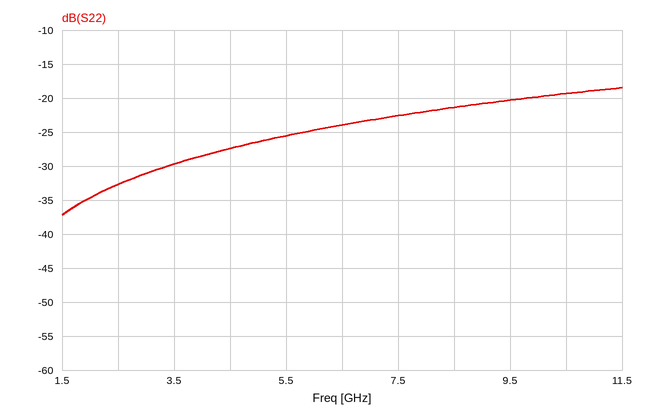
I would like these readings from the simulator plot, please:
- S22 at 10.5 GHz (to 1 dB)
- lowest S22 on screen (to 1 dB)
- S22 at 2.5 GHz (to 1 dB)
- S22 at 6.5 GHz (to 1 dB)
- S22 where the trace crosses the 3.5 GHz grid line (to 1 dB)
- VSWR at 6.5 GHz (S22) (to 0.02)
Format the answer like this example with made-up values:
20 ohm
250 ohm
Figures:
-19 dB
-37 dB
-33 dB
-24 dB
-30 dB
1.14
